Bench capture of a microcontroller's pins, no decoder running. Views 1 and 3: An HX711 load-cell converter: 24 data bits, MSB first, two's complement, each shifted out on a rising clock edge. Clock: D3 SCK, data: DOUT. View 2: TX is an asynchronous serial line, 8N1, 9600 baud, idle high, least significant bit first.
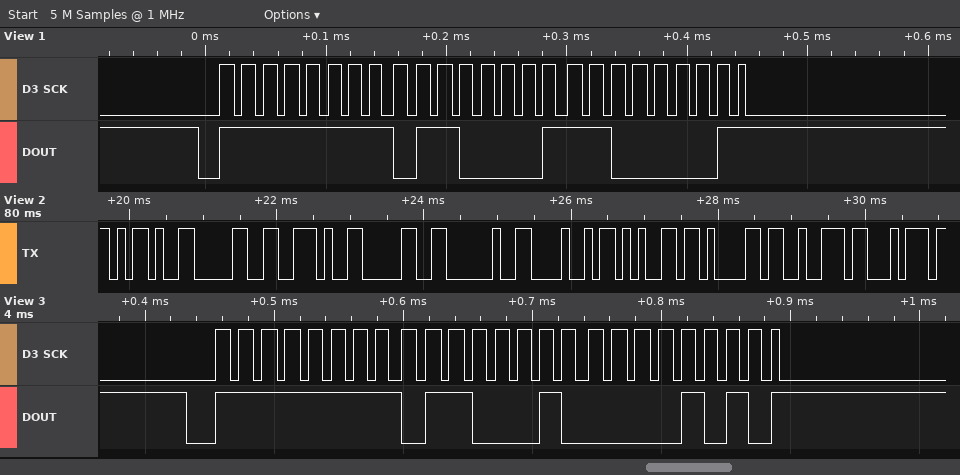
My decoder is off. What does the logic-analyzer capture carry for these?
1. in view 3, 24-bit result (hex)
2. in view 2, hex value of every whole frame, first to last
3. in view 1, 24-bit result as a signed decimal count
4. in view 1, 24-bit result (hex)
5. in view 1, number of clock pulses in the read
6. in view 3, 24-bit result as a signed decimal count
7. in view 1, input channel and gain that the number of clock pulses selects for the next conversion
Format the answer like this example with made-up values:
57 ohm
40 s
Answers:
0xFF620A
0x2D 0x30 0x2E 0x30 0x20 0x48 0x65 0x61 0x72 0x74
-40511
0xFF61C1
25
-40438
channel A, gain 128
